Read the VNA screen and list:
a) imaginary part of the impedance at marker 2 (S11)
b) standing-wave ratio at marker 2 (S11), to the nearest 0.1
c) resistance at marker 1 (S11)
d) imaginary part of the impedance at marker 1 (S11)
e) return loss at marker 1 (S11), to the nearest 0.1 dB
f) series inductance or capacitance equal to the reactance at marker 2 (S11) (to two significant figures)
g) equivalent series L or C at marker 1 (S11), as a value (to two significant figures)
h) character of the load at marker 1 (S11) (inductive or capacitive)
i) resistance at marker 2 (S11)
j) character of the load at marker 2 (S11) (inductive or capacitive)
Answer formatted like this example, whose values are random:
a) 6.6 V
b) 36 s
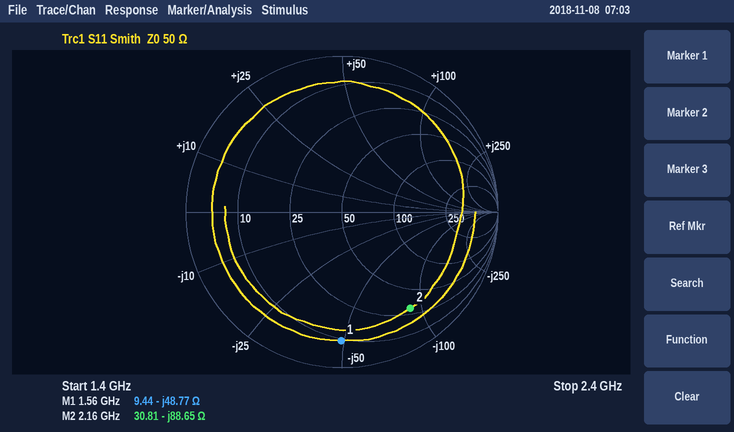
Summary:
a) -88.65 Ω
b) 7.2
c) 9.44 Ω
d) -48.77 Ω
e) 1.7 dB
f) 830 fF
g) 2.1 pF
h) capacitive
i) 30.81 Ω
j) capacitive
